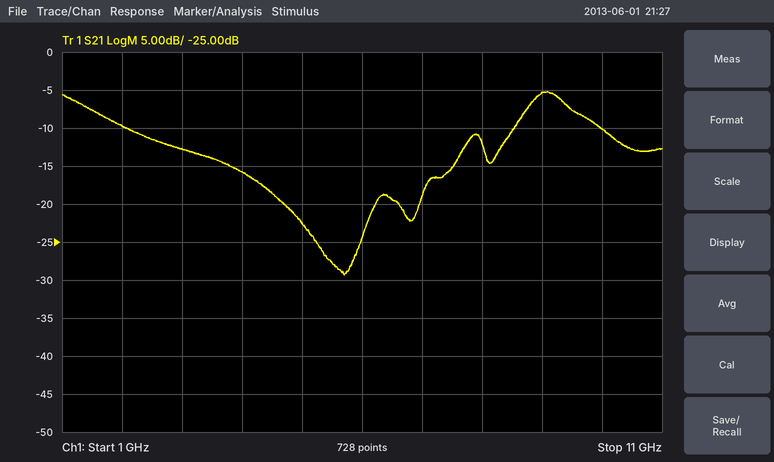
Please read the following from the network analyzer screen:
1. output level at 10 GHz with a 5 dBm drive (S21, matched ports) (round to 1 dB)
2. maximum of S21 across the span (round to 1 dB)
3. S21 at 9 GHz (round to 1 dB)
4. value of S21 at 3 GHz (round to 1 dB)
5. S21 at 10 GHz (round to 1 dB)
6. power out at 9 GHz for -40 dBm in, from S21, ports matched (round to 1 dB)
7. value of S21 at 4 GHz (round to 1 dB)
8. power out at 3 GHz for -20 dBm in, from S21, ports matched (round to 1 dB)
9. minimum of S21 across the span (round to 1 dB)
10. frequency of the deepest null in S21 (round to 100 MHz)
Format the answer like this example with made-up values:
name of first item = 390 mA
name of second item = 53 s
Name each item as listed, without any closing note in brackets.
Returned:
output level at 10 GHz with a 5 dBm drive (S21, matched ports) = -5 dBm
maximum of S21 across the span = -5 dB
S21 at 9 GHz = -5 dB
value of S21 at 3 GHz = -13 dB
S21 at 10 GHz = -10 dB
power out at 9 GHz for -40 dBm in, from S21, ports matched = -45 dBm
value of S21 at 4 GHz = -16 dB
power out at 3 GHz for -20 dBm in, from S21, ports matched = -33 dBm
minimum of S21 across the span = -29 dB
frequency of the deepest null in S21 = 5.7 GHz
